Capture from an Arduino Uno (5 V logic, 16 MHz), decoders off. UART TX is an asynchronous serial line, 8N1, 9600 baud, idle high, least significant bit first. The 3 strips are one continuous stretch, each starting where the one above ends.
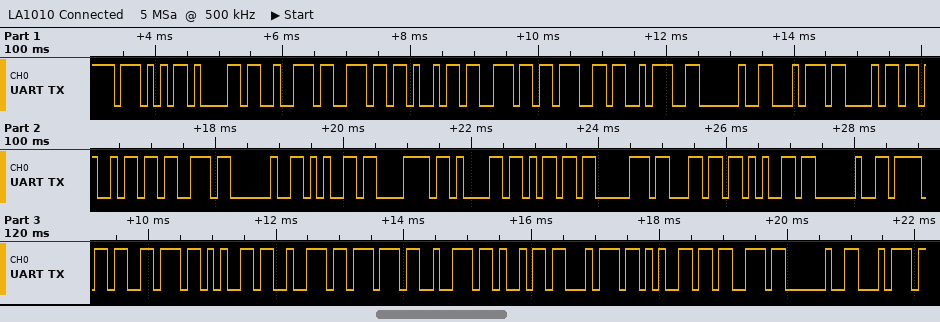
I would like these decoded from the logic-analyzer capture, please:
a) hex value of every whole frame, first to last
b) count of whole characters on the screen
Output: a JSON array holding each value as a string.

["57 61 72 6E 69 6E 67 3A 20 74 68 69 73 20 65 78 61 6D 70 6C 65 20 6F 76 65 72 77 72 69 74 65 73 20 74", "34"]
